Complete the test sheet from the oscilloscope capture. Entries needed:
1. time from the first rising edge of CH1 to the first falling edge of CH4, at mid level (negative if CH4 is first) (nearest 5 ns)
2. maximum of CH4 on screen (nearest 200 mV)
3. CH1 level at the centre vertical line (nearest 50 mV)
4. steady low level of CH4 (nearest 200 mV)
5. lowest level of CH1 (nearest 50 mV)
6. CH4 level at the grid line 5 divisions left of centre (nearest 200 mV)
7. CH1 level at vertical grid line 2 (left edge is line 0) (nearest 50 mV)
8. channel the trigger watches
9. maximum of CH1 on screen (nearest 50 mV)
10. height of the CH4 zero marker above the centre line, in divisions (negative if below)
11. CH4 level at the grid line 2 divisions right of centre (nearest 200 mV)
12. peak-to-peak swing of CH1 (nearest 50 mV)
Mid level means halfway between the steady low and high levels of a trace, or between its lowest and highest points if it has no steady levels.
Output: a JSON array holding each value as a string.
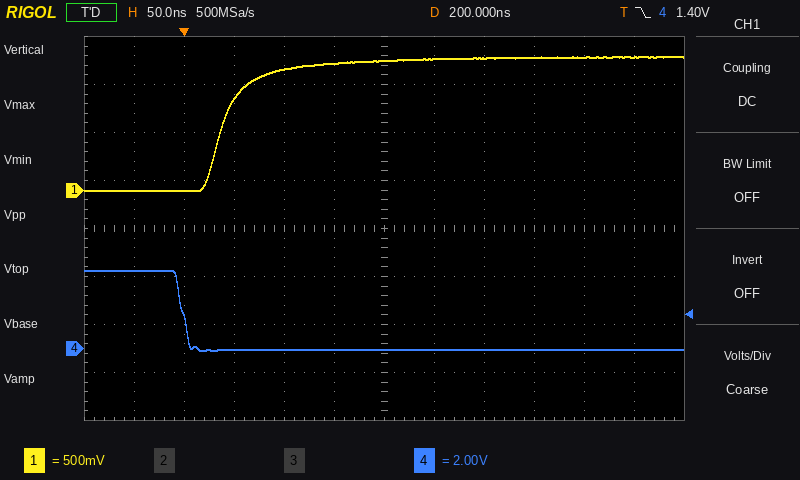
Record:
["-40 ns", "3.2 V", "1.35 V", "0.0 V", "0 mV", "3.2 V", "0 mV", "CH4", "1.40 V", "-2.5 div", "0.0 V", "1.40 V"]
